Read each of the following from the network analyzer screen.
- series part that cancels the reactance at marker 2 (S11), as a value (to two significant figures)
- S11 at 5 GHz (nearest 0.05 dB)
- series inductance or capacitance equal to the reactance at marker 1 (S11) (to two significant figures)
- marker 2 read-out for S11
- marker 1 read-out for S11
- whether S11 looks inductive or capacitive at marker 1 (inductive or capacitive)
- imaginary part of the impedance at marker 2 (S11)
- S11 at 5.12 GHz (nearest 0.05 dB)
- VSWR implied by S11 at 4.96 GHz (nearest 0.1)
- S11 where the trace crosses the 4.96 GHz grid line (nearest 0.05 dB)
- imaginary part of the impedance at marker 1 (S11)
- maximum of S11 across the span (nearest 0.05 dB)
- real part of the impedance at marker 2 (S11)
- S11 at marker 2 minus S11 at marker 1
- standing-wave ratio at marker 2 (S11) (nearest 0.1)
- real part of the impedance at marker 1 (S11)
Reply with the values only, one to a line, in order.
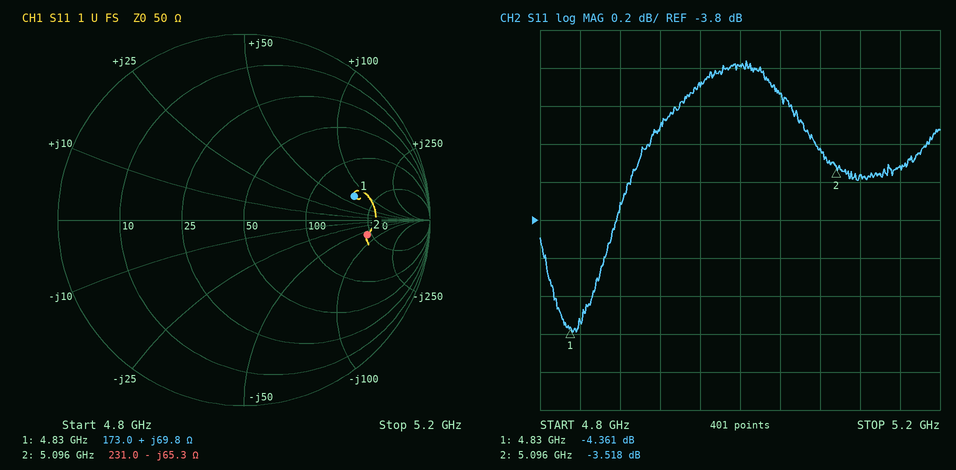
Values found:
2.0 nH
-3.00 dB
2.3 nH
-3.518 dB
-4.361 dB
inductive
-65.3 Ω
-3.55 dB
5.7
-3.10 dB
+69.8 Ω
-2.95 dB
231.0 Ω
0.843 dB
5.0
173.0 Ω
